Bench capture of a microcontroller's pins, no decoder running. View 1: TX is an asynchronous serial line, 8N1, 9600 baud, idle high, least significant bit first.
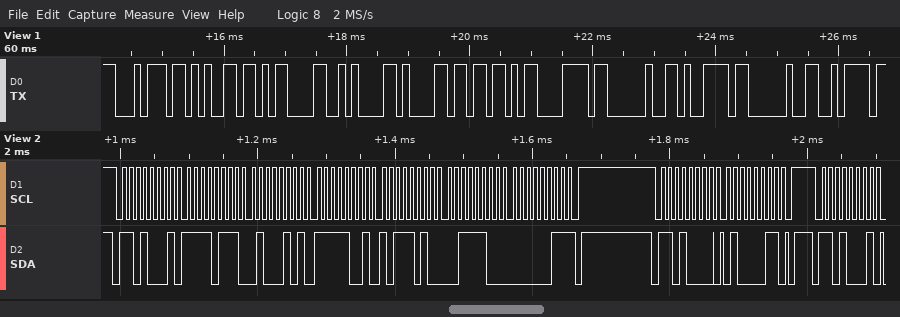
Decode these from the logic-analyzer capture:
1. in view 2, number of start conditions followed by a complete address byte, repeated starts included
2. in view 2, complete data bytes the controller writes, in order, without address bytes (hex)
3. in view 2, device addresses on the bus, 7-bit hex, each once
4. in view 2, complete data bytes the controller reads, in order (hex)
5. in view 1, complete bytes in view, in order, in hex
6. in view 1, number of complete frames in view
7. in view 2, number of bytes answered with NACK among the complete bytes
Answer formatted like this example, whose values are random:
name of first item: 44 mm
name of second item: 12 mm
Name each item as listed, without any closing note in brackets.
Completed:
in view 2, number of start conditions followed by a complete address byte, repeated starts included: 3
in view 2, complete data bytes the controller writes, in order, without address bytes: 43
in view 2, device addresses on the bus, 7-bit hex, each once: 0x68
in view 2, complete data bytes the controller reads, in order: F7 45 F9 BA 3C 03
in view 1, complete bytes in view, in order, in hex: 74 65 0D 0A 61 5B 78 20 79 20 7A
in view 1, number of complete frames in view: 11
in view 2, number of bytes answered with NACK among the complete bytes: 1
